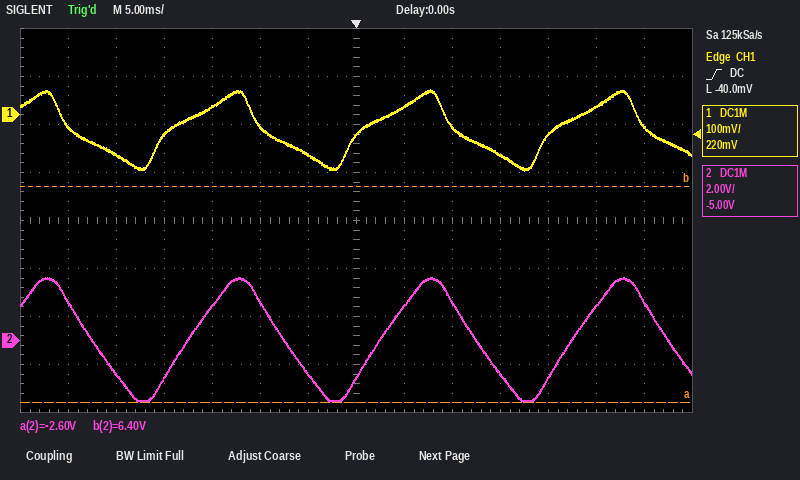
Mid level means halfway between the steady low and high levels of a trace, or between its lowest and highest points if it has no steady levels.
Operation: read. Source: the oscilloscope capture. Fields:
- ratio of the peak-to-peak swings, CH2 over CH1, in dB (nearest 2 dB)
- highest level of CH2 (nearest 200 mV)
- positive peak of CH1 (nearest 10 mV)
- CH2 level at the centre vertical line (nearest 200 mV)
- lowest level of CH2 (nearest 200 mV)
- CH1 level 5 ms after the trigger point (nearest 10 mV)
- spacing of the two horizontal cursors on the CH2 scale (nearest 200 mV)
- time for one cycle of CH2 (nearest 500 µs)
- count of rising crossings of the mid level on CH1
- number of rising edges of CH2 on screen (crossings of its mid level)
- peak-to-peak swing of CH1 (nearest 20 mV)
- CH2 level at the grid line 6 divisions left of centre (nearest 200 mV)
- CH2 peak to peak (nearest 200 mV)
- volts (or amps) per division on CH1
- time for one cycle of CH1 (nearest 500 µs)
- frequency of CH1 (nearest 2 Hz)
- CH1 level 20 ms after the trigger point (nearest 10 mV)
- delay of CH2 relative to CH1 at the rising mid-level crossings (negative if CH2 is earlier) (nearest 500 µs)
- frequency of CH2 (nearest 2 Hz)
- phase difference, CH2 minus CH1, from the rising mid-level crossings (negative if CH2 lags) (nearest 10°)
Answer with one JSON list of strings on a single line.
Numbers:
["30 dB", "2.6 V", "50 mV", "-1.6 V", "-2.6 V", "20 mV", "9.0 V", "20.0 ms", "3", "3", "160 mV", "1.6 V", "5.2 V", "100 mV", "20.0 ms", "50 Hz", "-40 mV", "+2.0 ms", "50 Hz", "-40°"]
